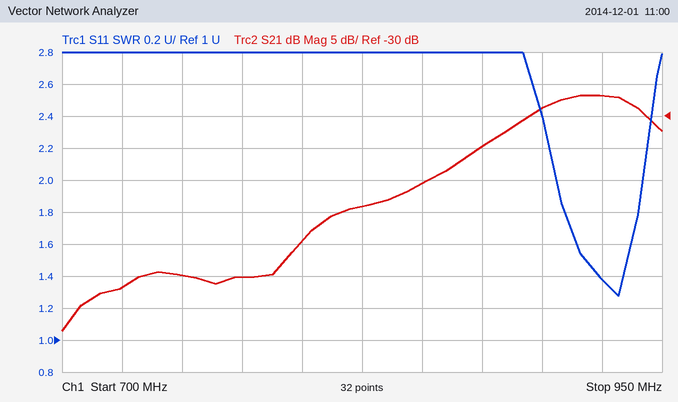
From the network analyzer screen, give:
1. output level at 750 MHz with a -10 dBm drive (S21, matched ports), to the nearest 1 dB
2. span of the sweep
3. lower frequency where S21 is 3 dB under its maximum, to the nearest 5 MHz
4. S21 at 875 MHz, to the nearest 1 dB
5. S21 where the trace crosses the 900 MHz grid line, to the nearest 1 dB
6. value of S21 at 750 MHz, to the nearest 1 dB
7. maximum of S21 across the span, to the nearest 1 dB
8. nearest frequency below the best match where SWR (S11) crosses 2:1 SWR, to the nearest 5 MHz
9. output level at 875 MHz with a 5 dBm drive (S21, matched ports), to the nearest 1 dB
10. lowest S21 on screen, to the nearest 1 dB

-65 dBm
250 MHz
895 MHz
-35 dB
-29 dB
-55 dB
-27 dB
905 MHz
-30 dBm
-64 dB
